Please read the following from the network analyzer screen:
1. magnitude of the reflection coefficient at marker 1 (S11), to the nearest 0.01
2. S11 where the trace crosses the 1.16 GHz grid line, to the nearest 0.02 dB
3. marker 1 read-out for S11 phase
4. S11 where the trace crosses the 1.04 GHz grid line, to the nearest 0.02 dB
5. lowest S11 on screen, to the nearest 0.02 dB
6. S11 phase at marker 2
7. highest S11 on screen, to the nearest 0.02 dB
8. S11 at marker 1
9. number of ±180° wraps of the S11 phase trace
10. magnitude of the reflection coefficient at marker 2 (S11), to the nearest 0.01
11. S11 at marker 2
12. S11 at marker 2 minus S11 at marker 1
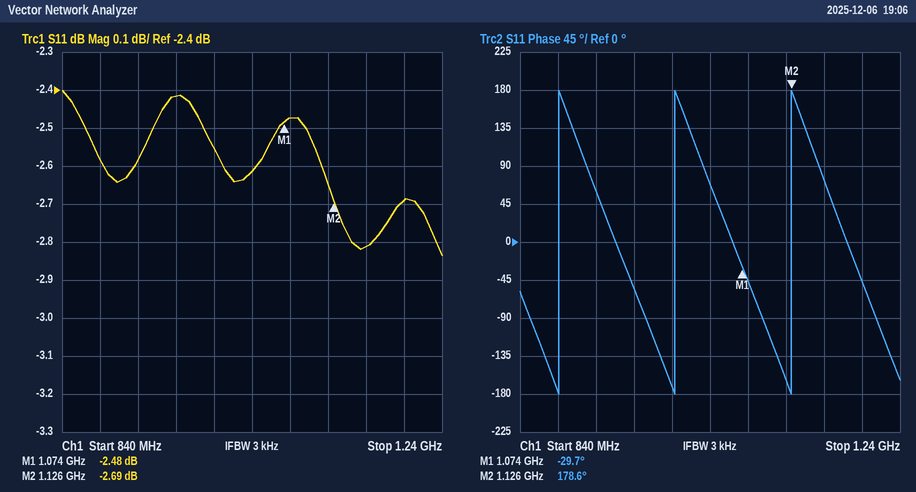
0.75
-2.82 dB
-29.7°
-2.62 dB
-2.84 dB
178.6°
-2.40 dB
-2.48 dB
3
0.73
-2.69 dB
-0.21 dB
